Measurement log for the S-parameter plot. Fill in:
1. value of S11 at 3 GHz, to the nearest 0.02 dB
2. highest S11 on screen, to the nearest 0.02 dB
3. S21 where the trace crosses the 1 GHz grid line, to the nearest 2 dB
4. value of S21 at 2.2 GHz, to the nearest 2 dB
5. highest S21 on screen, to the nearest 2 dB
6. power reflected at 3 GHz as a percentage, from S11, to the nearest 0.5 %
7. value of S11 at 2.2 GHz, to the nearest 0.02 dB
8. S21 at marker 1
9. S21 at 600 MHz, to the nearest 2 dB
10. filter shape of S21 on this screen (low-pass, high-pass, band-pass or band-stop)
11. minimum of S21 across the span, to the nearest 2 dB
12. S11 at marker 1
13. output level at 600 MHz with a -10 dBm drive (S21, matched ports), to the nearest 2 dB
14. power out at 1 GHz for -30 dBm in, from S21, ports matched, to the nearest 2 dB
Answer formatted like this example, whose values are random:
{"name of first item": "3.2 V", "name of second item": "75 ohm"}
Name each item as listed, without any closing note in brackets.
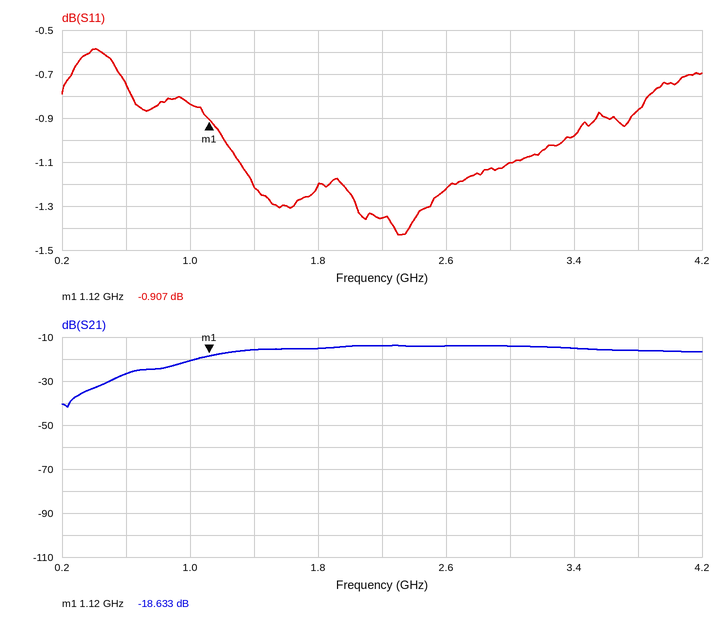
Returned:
{"value of S11 at 3 GHz, to the nearest 0.02 dB": "-1.10 dB", "highest S11 on screen, to the nearest 0.02 dB": "-0.58 dB", "S21 where the trace crosses the 1 GHz grid line, to the nearest 2 dB": "-20 dB", "value of S21 at 2.2 GHz, to the nearest 2 dB": "-14 dB", "highest S21 on screen, to the nearest 2 dB": "-14 dB", "power reflected at 3 GHz as a percentage, from S11, to the nearest 0.5 %": "77.5 %", "value of S11 at 2.2 GHz, to the nearest 0.02 dB": "-1.36 dB", "S21 at marker 1": "-18.633 dB", "S21 at 600 MHz, to the nearest 2 dB": "-26 dB", "filter shape of S21 on this screen": "high-pass", "minimum of S21 across the span, to the nearest 2 dB": "-42 dB", "S11 at marker 1": "-0.907 dB", "output level at 600 MHz with a -10 dBm drive (S21, matched ports), to the nearest 2 dB": "-36 dBm", "power out at 1 GHz for -30 dBm in, from S21, ports matched, to the nearest 2 dB": "-50 dBm"}
